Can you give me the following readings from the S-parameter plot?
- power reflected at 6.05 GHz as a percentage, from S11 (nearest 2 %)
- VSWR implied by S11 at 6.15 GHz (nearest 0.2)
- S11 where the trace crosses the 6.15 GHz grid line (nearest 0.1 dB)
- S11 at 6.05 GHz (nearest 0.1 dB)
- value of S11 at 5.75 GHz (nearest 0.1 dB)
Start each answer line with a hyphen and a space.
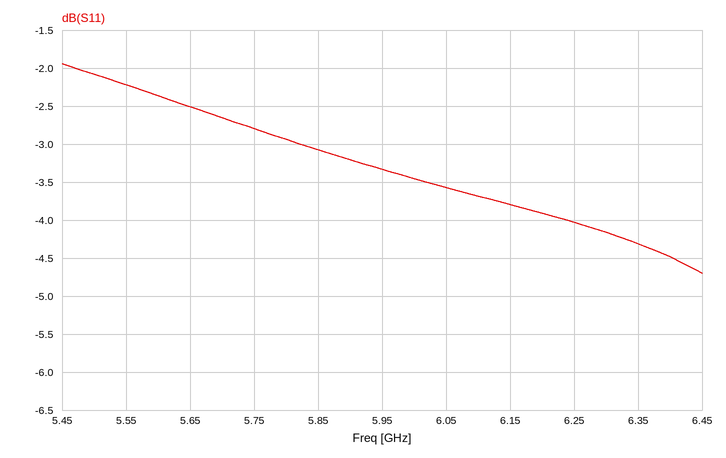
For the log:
- 44 %
- 4.6
- -3.8 dB
- -3.6 dB
- -2.8 dB
